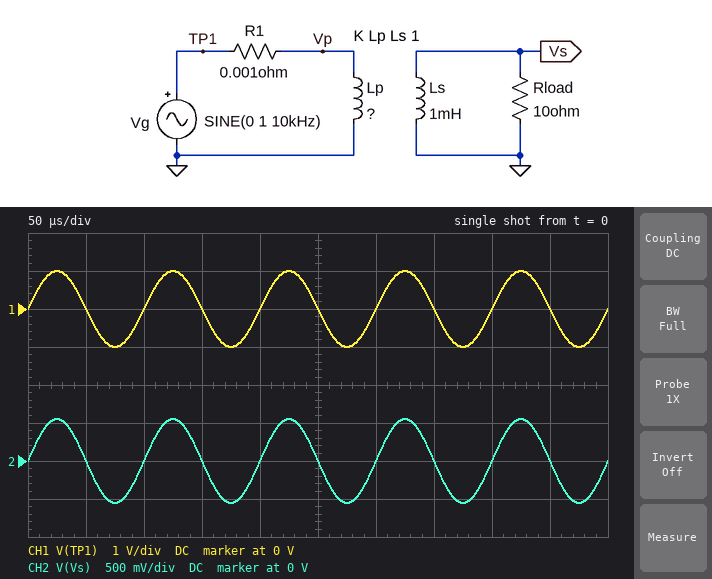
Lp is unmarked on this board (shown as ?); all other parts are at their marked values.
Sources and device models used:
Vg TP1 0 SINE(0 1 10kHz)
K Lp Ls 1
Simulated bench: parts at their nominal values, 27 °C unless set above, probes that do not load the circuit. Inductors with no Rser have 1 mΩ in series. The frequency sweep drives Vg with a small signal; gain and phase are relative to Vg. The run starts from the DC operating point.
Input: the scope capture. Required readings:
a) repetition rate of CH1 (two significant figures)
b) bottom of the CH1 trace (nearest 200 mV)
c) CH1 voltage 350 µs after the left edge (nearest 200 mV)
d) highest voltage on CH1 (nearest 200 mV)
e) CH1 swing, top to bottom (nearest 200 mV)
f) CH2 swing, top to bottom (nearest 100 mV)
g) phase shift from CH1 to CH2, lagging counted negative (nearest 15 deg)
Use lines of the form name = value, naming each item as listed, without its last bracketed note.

repetition rate of CH1 = 10 kHz
bottom of the CH1 trace = -1.0 V
CH1 voltage 350 µs after the left edge = 0 V
highest voltage on CH1 = 1.0 V
CH1 swing, top to bottom = 2.0 V
CH2 swing, top to bottom = 1.1 V
phase shift from CH1 to CH2, lagging counted negative = 0 deg
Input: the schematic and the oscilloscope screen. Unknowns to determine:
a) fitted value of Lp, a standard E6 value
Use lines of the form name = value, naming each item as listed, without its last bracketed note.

fitted value of Lp, a standard E6 value = 3.3 mH
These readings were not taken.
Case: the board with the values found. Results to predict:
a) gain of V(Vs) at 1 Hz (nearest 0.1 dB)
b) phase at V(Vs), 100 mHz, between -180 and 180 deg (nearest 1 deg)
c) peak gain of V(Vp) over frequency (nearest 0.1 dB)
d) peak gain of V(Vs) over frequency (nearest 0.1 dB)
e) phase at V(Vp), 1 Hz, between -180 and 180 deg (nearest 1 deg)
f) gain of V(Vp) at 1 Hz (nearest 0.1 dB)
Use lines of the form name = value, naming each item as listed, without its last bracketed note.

gain of V(Vs) at 1 Hz = -5.2 dB
phase at V(Vs), 100 mHz, between -180 and 180 deg = 44 deg
peak gain of V(Vp) over frequency = 0 dB
peak gain of V(Vs) over frequency = -5.2 dB
phase at V(Vp), 1 Hz, between -180 and 180 deg = 3 deg
gain of V(Vp) at 1 Hz = 0 dB
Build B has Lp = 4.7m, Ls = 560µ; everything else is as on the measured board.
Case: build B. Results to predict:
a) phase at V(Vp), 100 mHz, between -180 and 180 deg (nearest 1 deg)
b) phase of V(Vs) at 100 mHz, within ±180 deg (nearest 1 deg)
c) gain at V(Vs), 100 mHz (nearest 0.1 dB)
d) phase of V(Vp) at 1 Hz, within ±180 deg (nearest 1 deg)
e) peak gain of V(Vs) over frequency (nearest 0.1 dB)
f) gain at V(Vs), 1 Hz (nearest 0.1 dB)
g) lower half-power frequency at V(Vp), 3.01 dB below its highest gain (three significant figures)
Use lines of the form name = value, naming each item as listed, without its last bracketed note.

phase at V(Vp), 100 mHz, between -180 and 180 deg = 15 deg
phase of V(Vs) at 100 mHz, within ±180 deg = 34 deg
gain at V(Vs), 100 mHz = -10.9 dB
phase of V(Vp) at 1 Hz, within ±180 deg = 2 deg
peak gain of V(Vs) over frequency = -9.2 dB
gain at V(Vs), 1 Hz = -9.3 dB
lower half-power frequency at V(Vp), 3.01 dB below its highest gain = 47.9 mHz
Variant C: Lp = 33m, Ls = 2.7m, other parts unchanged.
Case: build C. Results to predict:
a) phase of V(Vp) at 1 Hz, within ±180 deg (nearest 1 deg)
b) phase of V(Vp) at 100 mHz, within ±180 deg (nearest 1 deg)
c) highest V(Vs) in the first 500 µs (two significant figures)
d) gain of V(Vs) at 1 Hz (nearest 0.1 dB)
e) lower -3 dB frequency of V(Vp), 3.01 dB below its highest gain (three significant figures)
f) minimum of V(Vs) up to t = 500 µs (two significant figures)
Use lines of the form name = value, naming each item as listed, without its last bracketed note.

phase of V(Vp) at 1 Hz, within ±180 deg = 0 deg
phase of V(Vp) at 100 mHz, within ±180 deg = 3 deg
highest V(Vs) in the first 500 µs = 290 mV
gain of V(Vs) at 1 Hz = -10.9 dB
lower -3 dB frequency of V(Vp), 3.01 dB below its highest gain = 6.82 mHz
minimum of V(Vs) up to t = 500 µs = -290 mV
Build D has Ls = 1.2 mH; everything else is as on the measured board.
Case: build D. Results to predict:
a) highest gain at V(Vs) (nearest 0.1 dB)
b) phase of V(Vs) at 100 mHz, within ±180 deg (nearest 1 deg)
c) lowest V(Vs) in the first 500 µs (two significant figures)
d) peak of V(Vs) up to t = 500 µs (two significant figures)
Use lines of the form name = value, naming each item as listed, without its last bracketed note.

highest gain at V(Vs) = -4.4 dB
phase of V(Vs) at 100 mHz, within ±180 deg = 44 deg
lowest V(Vs) in the first 500 µs = -600 mV
peak of V(Vs) up to t = 500 µs = 600 mV
